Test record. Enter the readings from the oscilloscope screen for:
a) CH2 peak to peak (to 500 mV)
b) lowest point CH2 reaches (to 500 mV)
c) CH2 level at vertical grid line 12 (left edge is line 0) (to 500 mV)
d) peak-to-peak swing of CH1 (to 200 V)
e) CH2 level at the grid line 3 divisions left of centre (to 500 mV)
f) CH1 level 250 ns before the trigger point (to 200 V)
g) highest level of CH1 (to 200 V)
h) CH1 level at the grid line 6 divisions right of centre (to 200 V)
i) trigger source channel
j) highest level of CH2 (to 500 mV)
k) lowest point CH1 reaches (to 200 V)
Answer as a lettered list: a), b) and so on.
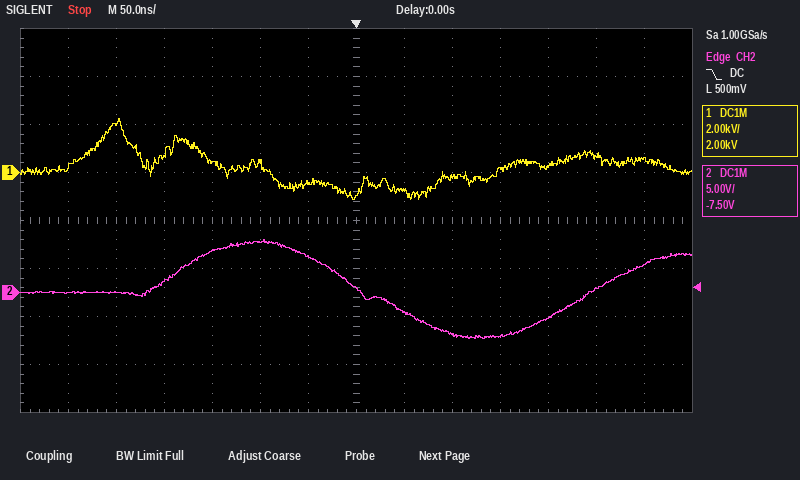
a) 10.5 V
b) -5.0 V
c) 500 mV
d) 3.4 kV
e) 4.5 V
f) 2.0 kV
g) 2.2 kV
h) 600 V
i) CH2
j) 5.5 V
k) -1.2 kV
